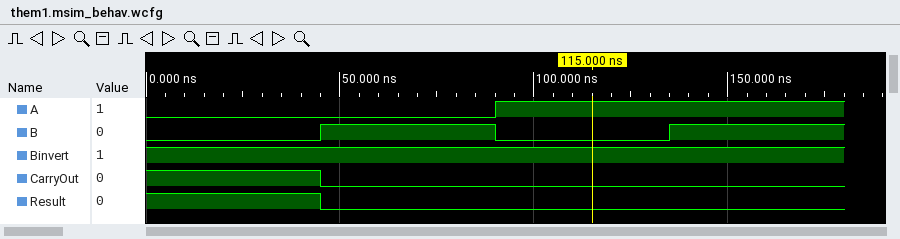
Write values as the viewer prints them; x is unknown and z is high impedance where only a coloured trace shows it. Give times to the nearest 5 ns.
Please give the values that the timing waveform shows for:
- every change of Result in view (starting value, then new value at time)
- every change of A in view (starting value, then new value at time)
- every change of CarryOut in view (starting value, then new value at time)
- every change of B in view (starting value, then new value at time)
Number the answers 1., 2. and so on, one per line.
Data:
1. 1, 0 at 45 ns
2. 0, 1 at 90 ns
3. 1, 0 at 45 ns
4. 0, 1 at 45 ns, 0 at 90 ns, 1 at 135 ns
